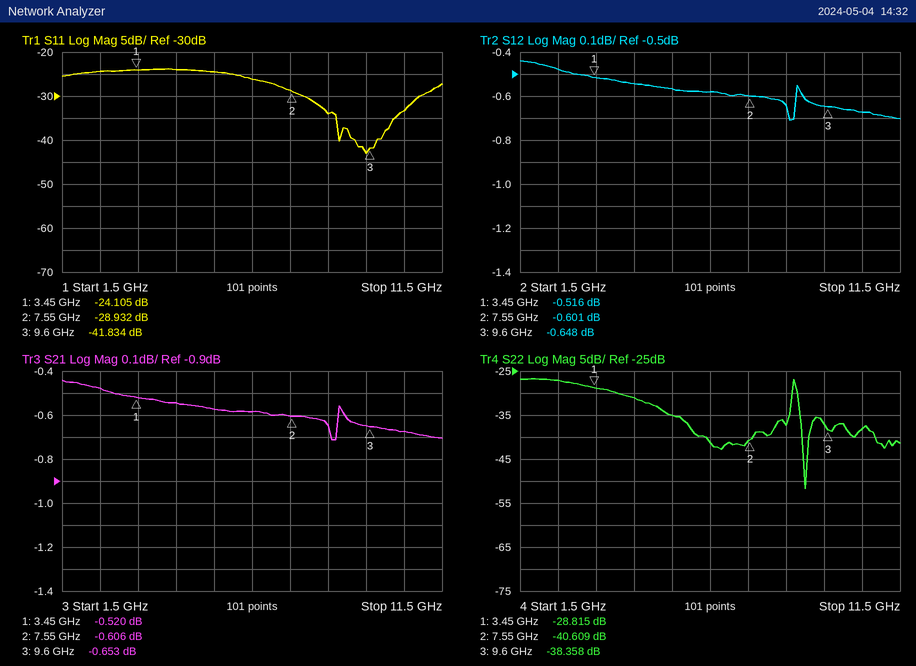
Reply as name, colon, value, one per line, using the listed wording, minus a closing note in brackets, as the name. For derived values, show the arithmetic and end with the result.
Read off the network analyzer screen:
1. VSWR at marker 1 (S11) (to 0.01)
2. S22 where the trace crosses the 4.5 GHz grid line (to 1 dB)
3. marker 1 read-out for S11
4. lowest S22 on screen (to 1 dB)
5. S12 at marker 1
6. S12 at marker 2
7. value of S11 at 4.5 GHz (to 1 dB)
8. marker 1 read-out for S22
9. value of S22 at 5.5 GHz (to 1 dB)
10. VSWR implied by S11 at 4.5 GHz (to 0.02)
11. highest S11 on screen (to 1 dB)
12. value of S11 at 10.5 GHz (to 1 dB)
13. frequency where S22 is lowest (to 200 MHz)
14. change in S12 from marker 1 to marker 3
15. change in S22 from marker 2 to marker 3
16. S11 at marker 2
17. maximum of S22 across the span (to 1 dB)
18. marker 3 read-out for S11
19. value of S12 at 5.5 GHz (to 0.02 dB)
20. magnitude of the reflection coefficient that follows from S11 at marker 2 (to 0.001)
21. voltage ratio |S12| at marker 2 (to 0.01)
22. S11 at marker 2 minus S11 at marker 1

VSWR at marker 1 (S11): (1 + 0.0623)/(1 − 0.0623) ≈ 1.13
S22 where the trace crosses the 4.5 GHz grid line: -31 dB
marker 1 read-out for S11: -24.105 dB
lowest S22 on screen: -52 dB
S12 at marker 1: -0.516 dB
S12 at marker 2: -0.601 dB
value of S11 at 4.5 GHz: -24 dB
marker 1 read-out for S22: -28.815 dB
value of S22 at 5.5 GHz: -35 dB
VSWR implied by S11 at 4.5 GHz: |Γ| = 10^(-24/20) = 0.0631; VSWR = (1 + 0.0631)/(1 − 0.0631) ≈ 1.13, so 1.14 to the nearest 0.02
highest S11 on screen: -24 dB
value of S11 at 10.5 GHz: -33 dB
frequency where S22 is lowest: 9.0 GHz
change in S12 from marker 1 to marker 3: -0.648 − (-0.516) = -0.132 dB
change in S22 from marker 2 to marker 3: -38.358 − (-40.609) = 2.251 dB
S11 at marker 2: -28.932 dB
maximum of S22 across the span: -27 dB
marker 3 read-out for S11: -41.834 dB
value of S12 at 5.5 GHz: -0.56 dB
magnitude of the reflection coefficient that follows from S11 at marker 2: 10^(-28.932/20) ≈ 0.036
voltage ratio |S12| at marker 2: 10^(-0.601/20) ≈ 0.93
S11 at marker 2 minus S11 at marker 1: -28.932 − (-24.105) = -4.827 dB
